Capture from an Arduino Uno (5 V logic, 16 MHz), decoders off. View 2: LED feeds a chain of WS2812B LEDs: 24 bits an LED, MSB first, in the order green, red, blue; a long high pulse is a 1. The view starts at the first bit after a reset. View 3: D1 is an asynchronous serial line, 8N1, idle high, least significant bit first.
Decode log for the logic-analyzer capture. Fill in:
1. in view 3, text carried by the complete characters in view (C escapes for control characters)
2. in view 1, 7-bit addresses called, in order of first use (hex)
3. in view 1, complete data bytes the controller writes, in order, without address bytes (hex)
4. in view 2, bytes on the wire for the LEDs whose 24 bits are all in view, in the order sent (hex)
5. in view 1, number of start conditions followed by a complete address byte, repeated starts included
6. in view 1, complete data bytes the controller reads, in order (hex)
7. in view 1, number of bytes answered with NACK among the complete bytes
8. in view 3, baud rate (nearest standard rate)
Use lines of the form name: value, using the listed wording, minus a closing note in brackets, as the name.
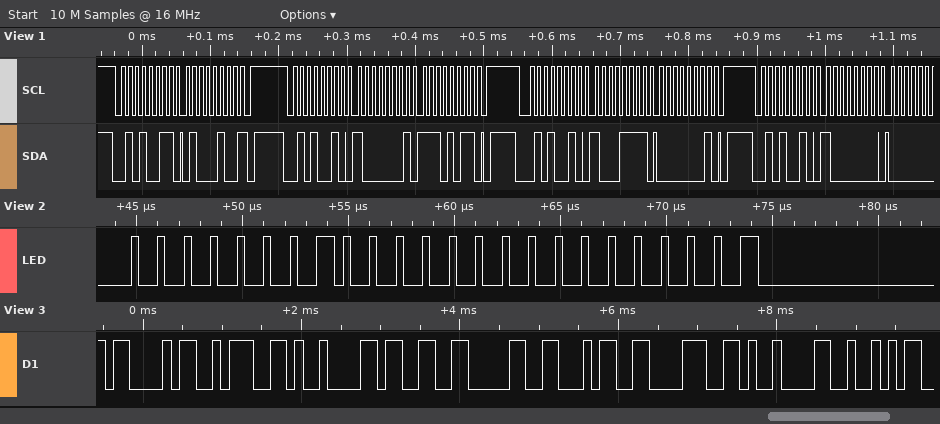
in view 3, text carried by the complete characters in view: "C:\t3048\tR"
in view 1, 7-bit addresses called, in order of first use: 0x29
in view 1, complete data bytes the controller writes, in order, without address bytes: 81 EB 8F 01 80
in view 2, bytes on the wire for the LEDs whose 24 bits are all in view, in the order sent: 01 00 01
in view 1, number of start conditions followed by a complete address byte, repeated starts included: 4
in view 1, complete data bytes the controller reads, in order: 44
in view 1, number of bytes answered with NACK among the complete bytes: 1
in view 3, baud rate: 9600 baud
